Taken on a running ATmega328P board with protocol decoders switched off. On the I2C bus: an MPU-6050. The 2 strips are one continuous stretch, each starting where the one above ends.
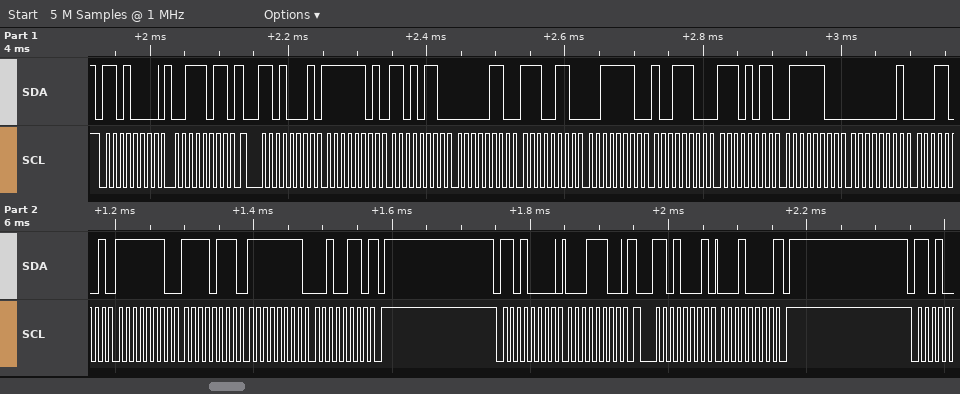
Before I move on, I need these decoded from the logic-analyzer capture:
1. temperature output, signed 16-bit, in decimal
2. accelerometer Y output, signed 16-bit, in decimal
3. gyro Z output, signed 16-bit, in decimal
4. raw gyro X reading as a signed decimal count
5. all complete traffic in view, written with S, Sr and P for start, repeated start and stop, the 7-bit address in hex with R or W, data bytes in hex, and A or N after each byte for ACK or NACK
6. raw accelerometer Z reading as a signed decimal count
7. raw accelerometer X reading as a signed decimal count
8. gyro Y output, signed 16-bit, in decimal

-5252
1766
-218
281
S 68W A 3B A Sr 68R A FD A D6 A 06 A E6 A 3E A 9C A EB A 7C A 01 A 19 A FE A F7 A FF A 26 N P S 68W A 1C A Sr 68R A 10 N P
16028
-554
-265
